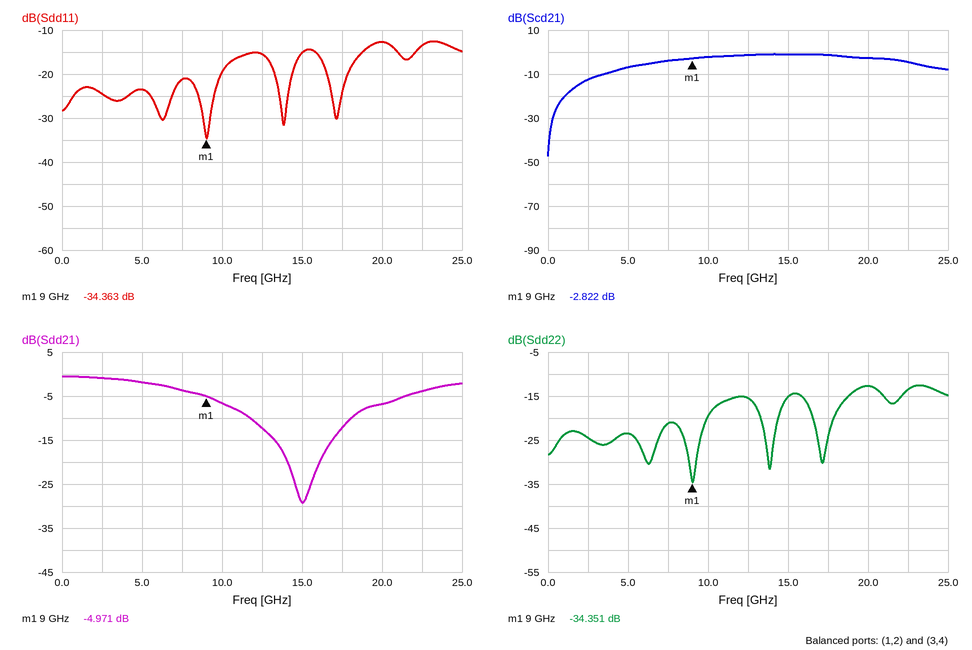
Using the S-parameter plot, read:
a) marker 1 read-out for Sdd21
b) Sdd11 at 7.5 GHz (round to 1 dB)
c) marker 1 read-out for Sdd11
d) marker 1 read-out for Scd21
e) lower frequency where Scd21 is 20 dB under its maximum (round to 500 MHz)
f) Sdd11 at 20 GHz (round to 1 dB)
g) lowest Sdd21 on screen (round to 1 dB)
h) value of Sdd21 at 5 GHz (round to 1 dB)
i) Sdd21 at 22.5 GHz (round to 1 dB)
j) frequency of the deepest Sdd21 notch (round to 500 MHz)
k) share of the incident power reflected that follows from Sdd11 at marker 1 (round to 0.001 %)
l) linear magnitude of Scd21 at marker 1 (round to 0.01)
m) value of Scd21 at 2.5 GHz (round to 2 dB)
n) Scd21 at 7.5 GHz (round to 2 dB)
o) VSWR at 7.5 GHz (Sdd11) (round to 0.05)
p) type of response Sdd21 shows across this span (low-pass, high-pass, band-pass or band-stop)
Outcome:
-4.971 dB
-21 dB
-34.363 dB
-2.822 dB
1.0 GHz
-13 dB
-29 dB
-2 dB
-4 dB
15.0 GHz
0.037 %
0.72
-12 dB
-4 dB
1.20
band-stop
